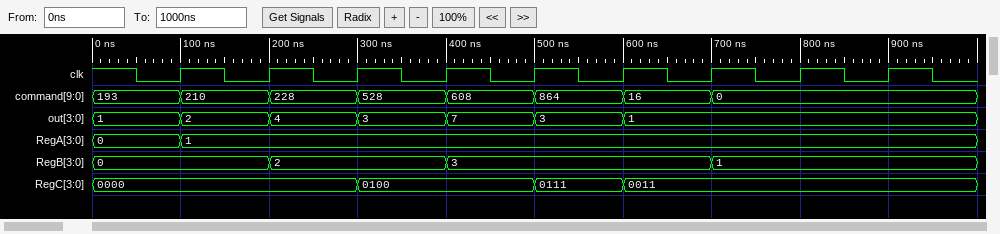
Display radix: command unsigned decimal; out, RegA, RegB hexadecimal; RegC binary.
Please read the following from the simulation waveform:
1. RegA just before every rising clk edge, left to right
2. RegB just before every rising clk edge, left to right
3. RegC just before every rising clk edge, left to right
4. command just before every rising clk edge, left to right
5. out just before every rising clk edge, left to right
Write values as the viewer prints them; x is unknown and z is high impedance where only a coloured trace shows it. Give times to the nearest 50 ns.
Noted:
0, 1, 1, 1, 1, 1, 1, 1, 1
0, 0, 2, 2, 3, 3, 3, 1, 1
0000, 0000, 0000, 0100, 0100, 0111, 0011, 0011, 0011
193, 210, 228, 528, 608, 864, 16, 0, 0
1, 2, 4, 3, 7, 3, 1, 1, 1
